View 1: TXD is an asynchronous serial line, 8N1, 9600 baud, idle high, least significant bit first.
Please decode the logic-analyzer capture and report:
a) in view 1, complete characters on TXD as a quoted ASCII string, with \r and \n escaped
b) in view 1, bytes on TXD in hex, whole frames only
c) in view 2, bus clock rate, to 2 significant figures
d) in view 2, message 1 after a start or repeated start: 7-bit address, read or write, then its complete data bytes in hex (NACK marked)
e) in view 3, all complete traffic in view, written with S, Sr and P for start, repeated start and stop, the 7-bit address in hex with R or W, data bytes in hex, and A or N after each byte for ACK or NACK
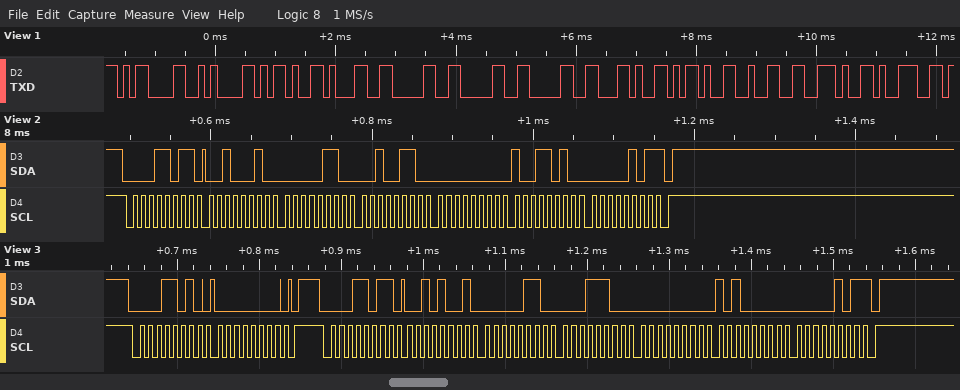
"\r\n-1000,-2.9"
0D 0A 2D 31 30 30 30 2C 2D 32 2E 39
100 kHz
0x0D read: 22 06 26 00 9A 05 NACK
S 0DW A 00 A P S 0DR A 29 A 06 A 1C A 00 A A0 A 05 N P
